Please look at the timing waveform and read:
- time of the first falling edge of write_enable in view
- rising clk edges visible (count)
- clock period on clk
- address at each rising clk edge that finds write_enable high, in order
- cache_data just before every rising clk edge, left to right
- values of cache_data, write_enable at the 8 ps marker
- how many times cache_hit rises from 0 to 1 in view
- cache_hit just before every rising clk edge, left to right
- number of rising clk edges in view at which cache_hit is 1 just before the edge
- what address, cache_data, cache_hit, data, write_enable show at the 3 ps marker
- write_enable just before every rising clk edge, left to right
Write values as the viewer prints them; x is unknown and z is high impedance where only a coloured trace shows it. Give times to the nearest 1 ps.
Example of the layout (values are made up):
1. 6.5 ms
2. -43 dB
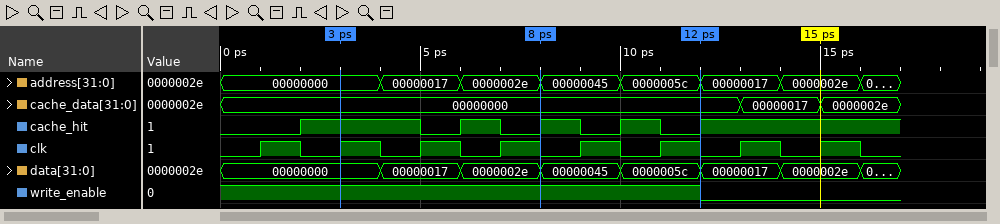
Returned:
1. 12 ps
2. 8
3. 2 ps
4. 00000000, 00000000, 00000017, 0000002e, 00000045, 0000005c
5. 00000000, 00000000, 00000000, 00000000, 00000000, 00000000, 00000000, 00000017
6. cache_data=00000000, write_enable=1
7. 5
8. 0 1 1 1 1 1 1 1
9. 7
10. address=00000000, cache_data=00000000, cache_hit=1, data=00000000, write_enable=1
11. 1 1 1 1 1 1 0 0
